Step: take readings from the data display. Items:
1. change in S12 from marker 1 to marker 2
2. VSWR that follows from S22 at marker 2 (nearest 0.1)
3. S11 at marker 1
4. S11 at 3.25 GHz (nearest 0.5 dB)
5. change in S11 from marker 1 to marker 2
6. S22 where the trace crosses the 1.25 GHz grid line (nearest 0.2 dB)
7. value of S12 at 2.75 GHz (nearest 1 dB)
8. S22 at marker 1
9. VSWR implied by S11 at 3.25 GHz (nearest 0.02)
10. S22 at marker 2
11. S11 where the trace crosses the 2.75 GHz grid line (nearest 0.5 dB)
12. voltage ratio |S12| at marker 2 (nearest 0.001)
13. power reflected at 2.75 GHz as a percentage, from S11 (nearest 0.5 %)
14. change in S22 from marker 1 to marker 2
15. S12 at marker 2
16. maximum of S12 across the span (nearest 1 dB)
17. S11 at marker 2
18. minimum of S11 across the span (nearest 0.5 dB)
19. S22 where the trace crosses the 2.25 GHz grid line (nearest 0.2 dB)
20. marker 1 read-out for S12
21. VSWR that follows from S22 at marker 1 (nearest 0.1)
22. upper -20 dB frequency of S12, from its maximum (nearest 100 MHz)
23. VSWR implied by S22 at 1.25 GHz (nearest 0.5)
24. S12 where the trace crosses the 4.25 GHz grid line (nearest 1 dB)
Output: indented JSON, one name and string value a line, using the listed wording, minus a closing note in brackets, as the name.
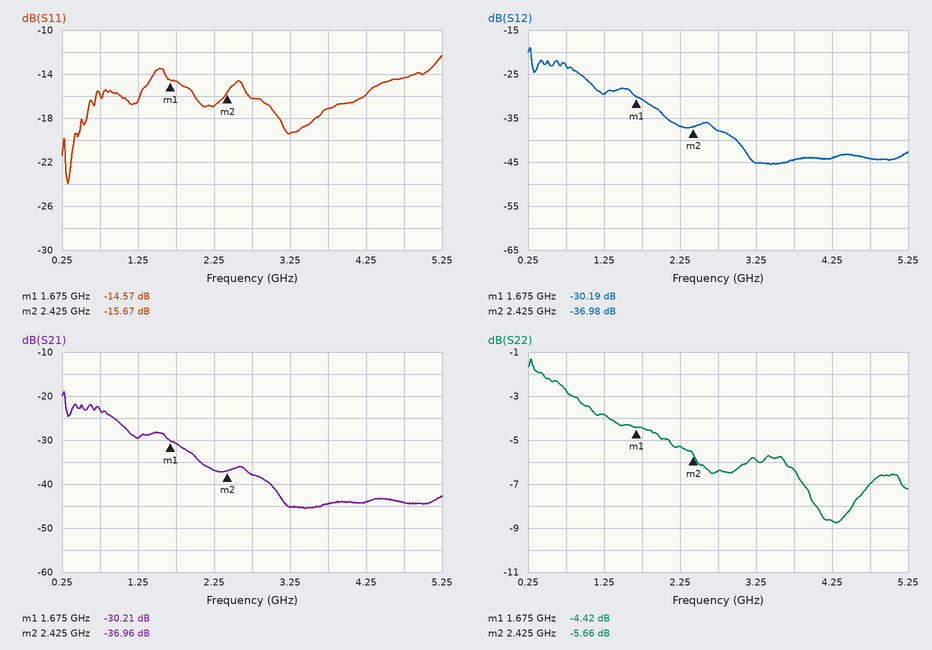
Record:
{
  "change in S12 from marker 1 to marker 2": "-6.79 dB",
  "VSWR that follows from S22 at marker 2": "3.2",
  "S11 at marker 1": "-14.57 dB",
  "S11 at 3.25 GHz": "-19.5 dB",
  "change in S11 from marker 1 to marker 2": "-1.10 dB",
  "S22 where the trace crosses the 1.25 GHz grid line": "-3.8 dB",
  "value of S12 at 2.75 GHz": "-38 dB",
  "S22 at marker 1": "-4.42 dB",
  "VSWR implied by S11 at 3.25 GHz": "1.24",
  "S22 at marker 2": "-5.66 dB",
  "S11 where the trace crosses the 2.75 GHz grid line": "-16.0 dB",
  "voltage ratio |S12| at marker 2": "0.014",
  "power reflected at 2.75 GHz as a percentage, from S11": "2.5 %",
  "change in S22 from marker 1 to marker 2": "-1.24 dB",
  "S12 at marker 2": "-36.98 dB",
  "maximum of S12 across the span": "-19 dB",
  "S11 at marker 2": "-15.67 dB",
  "minimum of S11 across the span": "-24.0 dB",
  "S22 where the trace crosses the 2.25 GHz grid line": "-5.2 dB",
  "marker 1 read-out for S12": "-30.19 dB",
  "VSWR that follows from S22 at marker 1": "4.0",
  "upper -20 dB frequency of S12, from its maximum": "2.9 GHz",
  "VSWR implied by S22 at 1.25 GHz": "4.5",
  "S12 where the trace crosses the 4.25 GHz grid line": "-44 dB"
}
